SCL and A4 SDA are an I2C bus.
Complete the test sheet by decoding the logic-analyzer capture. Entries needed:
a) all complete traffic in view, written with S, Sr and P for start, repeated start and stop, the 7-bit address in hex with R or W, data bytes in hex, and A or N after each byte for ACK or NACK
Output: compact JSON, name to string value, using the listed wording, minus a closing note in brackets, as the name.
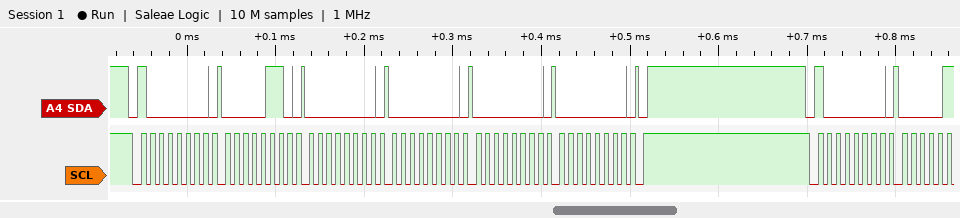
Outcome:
{"all complete traffic in view, written with S, Sr and P for start, repeated start and stop, the 7-bit address in hex with R or W, data bytes in hex, and A or N after each byte for ACK or NACK": "S 40W A 06 A 00 A 00 A 00 A 00 A P S 40W A"}
